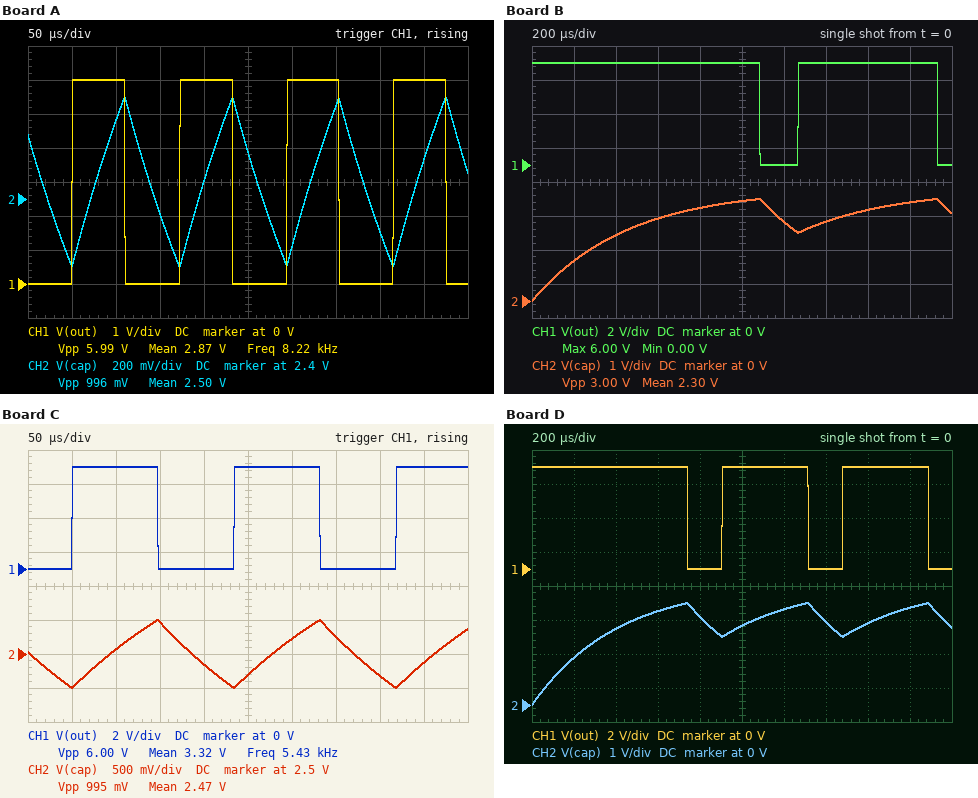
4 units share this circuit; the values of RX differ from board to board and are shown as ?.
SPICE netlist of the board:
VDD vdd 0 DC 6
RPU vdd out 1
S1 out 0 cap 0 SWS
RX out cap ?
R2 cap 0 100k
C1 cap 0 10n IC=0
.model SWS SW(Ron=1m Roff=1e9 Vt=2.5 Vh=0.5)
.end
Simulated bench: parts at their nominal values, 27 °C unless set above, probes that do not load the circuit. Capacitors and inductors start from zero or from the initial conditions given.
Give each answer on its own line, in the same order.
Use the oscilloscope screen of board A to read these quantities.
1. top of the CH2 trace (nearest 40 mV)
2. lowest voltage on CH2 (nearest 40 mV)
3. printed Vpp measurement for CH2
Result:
3.00 V
2.00 V
996 mV
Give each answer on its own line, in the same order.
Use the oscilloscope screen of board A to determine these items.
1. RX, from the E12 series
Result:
18 kΩ
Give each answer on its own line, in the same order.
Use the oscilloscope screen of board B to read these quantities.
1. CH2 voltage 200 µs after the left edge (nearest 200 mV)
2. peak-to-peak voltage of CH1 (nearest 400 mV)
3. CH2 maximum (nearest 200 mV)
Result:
1.2 V
6.0 V
3.0 V
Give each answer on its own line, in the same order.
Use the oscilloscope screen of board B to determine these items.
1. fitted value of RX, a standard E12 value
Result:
82 kΩ
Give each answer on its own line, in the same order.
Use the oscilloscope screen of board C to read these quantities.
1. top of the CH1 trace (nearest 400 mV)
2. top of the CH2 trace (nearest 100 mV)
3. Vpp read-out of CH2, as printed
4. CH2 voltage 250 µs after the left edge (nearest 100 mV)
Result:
6.0 V
3.0 V
995 mV
2.2 V
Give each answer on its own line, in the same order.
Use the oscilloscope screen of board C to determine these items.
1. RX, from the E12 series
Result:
27 kΩ
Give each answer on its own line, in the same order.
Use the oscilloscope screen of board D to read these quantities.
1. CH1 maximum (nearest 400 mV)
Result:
6.0 V
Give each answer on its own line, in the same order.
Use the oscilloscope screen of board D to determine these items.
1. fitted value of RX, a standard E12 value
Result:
68 kΩ
